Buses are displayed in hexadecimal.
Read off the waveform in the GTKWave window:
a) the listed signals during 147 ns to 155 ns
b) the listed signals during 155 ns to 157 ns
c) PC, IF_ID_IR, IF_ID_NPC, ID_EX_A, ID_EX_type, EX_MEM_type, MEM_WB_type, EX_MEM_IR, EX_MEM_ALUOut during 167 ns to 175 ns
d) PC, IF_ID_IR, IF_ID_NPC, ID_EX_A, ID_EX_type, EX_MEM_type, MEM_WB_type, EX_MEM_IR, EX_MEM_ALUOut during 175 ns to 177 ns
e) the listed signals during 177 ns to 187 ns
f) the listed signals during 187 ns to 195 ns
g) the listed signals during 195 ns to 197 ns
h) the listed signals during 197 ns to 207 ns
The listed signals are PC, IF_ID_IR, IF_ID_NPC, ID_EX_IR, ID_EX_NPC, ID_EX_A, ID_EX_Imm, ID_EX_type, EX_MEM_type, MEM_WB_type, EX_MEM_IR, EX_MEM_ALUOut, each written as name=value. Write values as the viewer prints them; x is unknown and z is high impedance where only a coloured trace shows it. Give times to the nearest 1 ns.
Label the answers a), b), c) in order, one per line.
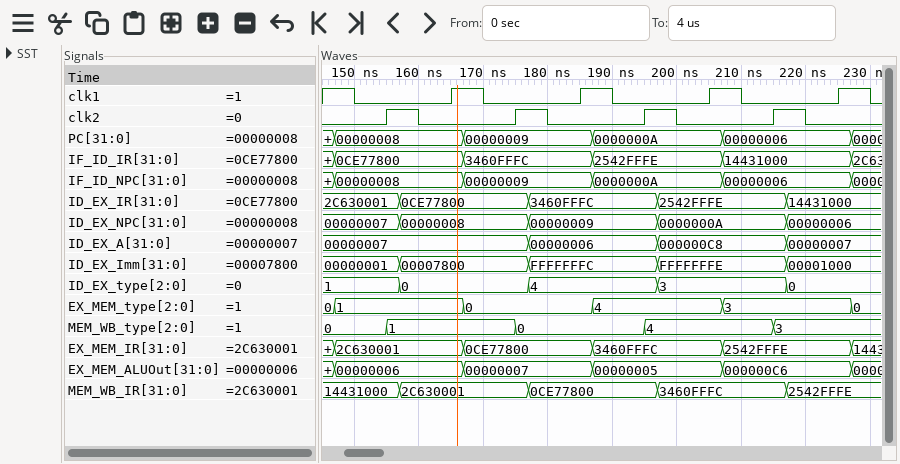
a) PC=00000008, IF_ID_IR=0CE77800, IF_ID_NPC=00000008, ID_EX_IR=2C630001, ID_EX_NPC=00000007, ID_EX_A=00000007, ID_EX_Imm=00000001, ID_EX_type=1, EX_MEM_type=1, MEM_WB_type=0, EX_MEM_IR=2C630001, EX_MEM_ALUOut=00000006
b) PC=00000008, IF_ID_IR=0CE77800, IF_ID_NPC=00000008, ID_EX_IR=2C630001, ID_EX_NPC=00000007, ID_EX_A=00000007, ID_EX_Imm=00000001, ID_EX_type=1, EX_MEM_type=1, MEM_WB_type=1, EX_MEM_IR=2C630001, EX_MEM_ALUOut=00000006
c) PC=00000009, IF_ID_IR=3460FFFC, IF_ID_NPC=00000009, ID_EX_A=00000007, ID_EX_type=0, EX_MEM_type=0, MEM_WB_type=1, EX_MEM_IR=0CE77800, EX_MEM_ALUOut=00000007
d) PC=00000009, IF_ID_IR=3460FFFC, IF_ID_NPC=00000009, ID_EX_A=00000007, ID_EX_type=0, EX_MEM_type=0, MEM_WB_type=0, EX_MEM_IR=0CE77800, EX_MEM_ALUOut=00000007
e) PC=00000009, IF_ID_IR=3460FFFC, IF_ID_NPC=00000009, ID_EX_IR=3460FFFC, ID_EX_NPC=00000009, ID_EX_A=00000006, ID_EX_Imm=FFFFFFFC, ID_EX_type=4, EX_MEM_type=0, MEM_WB_type=0, EX_MEM_IR=0CE77800, EX_MEM_ALUOut=00000007
f) PC=0000000A, IF_ID_IR=2542FFFE, IF_ID_NPC=0000000A, ID_EX_IR=3460FFFC, ID_EX_NPC=00000009, ID_EX_A=00000006, ID_EX_Imm=FFFFFFFC, ID_EX_type=4, EX_MEM_type=4, MEM_WB_type=0, EX_MEM_IR=3460FFFC, EX_MEM_ALUOut=00000005
g) PC=0000000A, IF_ID_IR=2542FFFE, IF_ID_NPC=0000000A, ID_EX_IR=3460FFFC, ID_EX_NPC=00000009, ID_EX_A=00000006, ID_EX_Imm=FFFFFFFC, ID_EX_type=4, EX_MEM_type=4, MEM_WB_type=4, EX_MEM_IR=3460FFFC, EX_MEM_ALUOut=00000005
h) PC=0000000A, IF_ID_IR=2542FFFE, IF_ID_NPC=0000000A, ID_EX_IR=2542FFFE, ID_EX_NPC=0000000A, ID_EX_A=000000C8, ID_EX_Imm=FFFFFFFE, ID_EX_type=3, EX_MEM_type=4, MEM_WB_type=4, EX_MEM_IR=3460FFFC, EX_MEM_ALUOut=00000005
